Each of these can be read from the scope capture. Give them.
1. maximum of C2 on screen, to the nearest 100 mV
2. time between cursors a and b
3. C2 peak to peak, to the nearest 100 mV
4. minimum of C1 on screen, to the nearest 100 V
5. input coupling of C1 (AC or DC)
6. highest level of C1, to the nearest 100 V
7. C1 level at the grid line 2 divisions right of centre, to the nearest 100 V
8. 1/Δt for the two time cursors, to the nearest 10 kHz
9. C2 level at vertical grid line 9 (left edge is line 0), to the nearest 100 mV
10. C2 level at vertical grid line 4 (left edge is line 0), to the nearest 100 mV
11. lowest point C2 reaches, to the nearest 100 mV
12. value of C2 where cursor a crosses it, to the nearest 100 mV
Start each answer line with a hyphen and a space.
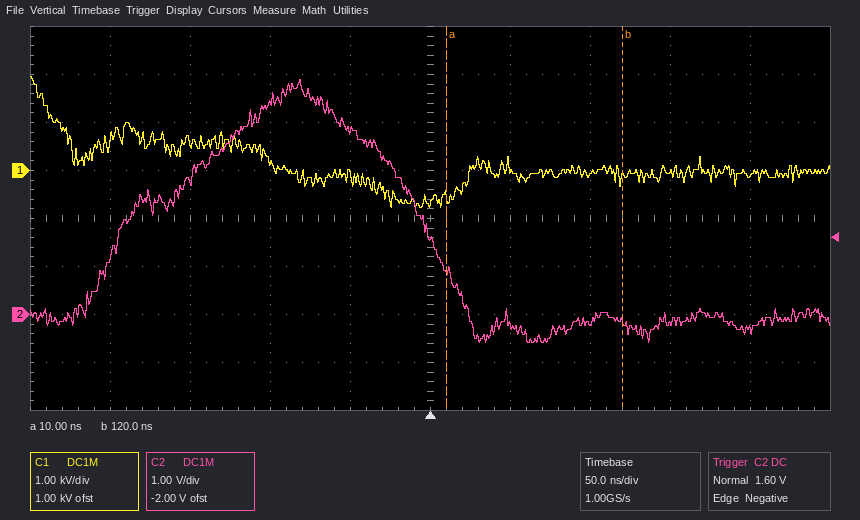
- 4.9 V
- 110 ns
- 5.5 V
- -800 V
- DC
- 2.0 kV
- -100 V
- 9.09 MHz
- -300 mV
- 3.8 V
- -600 mV
- 900 mV
